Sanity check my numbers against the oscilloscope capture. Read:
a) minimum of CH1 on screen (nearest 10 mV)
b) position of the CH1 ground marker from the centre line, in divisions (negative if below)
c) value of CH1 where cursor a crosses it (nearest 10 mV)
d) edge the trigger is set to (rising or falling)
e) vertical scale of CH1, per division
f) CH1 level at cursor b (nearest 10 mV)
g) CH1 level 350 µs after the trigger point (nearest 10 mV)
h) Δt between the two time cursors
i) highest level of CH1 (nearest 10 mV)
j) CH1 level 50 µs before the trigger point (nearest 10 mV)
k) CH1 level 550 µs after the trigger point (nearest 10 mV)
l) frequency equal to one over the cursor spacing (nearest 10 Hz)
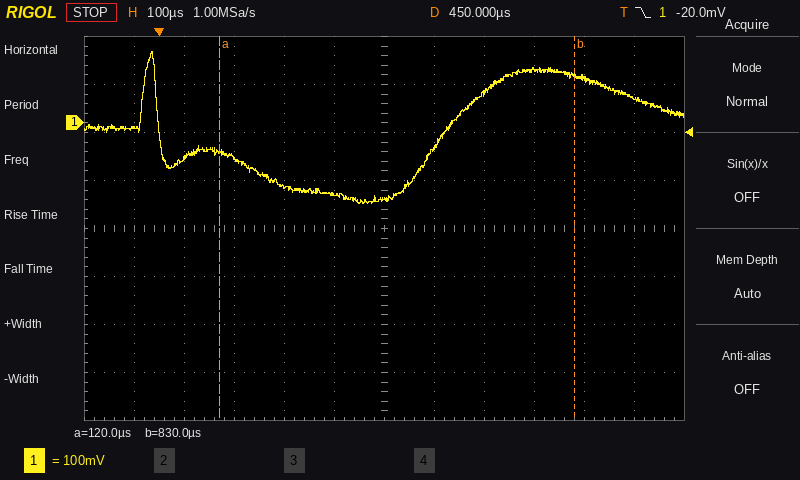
-170 mV
+2.2 div
-60 mV
falling
100 mV
100 mV
-150 mV
710 µs
150 mV
-10 mV
-50 mV
1.41 kHz
